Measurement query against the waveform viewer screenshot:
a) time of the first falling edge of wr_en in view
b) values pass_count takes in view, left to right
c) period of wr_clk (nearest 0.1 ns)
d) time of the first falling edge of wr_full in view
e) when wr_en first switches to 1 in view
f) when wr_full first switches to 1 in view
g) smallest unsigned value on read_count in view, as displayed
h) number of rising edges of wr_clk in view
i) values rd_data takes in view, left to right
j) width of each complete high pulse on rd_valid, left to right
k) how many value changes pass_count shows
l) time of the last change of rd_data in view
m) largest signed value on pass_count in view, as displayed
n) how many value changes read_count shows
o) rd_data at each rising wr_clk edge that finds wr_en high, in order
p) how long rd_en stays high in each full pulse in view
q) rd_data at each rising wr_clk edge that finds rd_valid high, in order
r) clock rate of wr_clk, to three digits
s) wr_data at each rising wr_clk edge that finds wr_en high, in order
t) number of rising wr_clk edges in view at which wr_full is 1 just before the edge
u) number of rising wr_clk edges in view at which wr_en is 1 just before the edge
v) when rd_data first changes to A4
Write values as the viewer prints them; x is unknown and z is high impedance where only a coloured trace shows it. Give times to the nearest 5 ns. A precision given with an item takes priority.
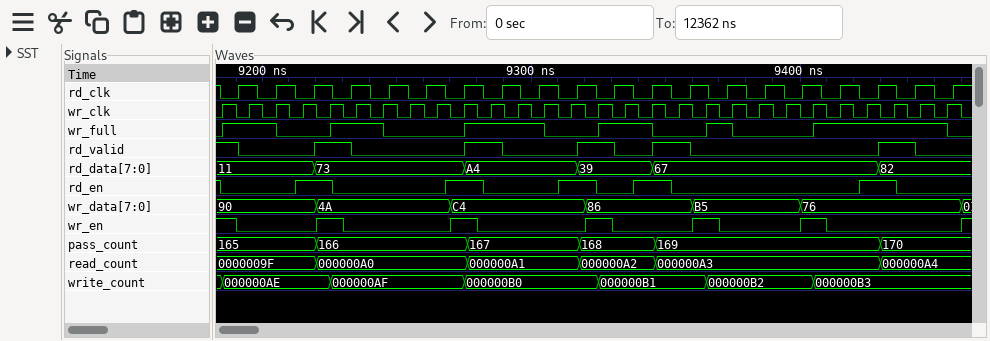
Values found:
9190 ns
165, 166, 167, 168, 169, 170
10 ns
9205 ns
9220 ns
9185 ns
0000009F
28
11, 73, A4, 39, 67, 82
15 ns, 15 ns, 15 ns, 15 ns, 15 ns
5
9430 ns
170
5
11, 73, 73, 39, 67, 67
15 ns, 15 ns, 15 ns, 15 ns, 15 ns
11, 73, A4, 39, 67, 82
100 MHz
90, 4A, C4, 86, B5, 76
15
6
9275 ns
